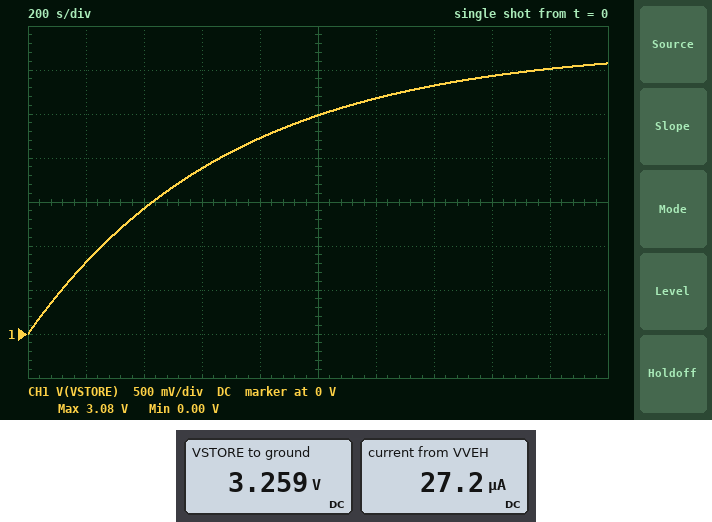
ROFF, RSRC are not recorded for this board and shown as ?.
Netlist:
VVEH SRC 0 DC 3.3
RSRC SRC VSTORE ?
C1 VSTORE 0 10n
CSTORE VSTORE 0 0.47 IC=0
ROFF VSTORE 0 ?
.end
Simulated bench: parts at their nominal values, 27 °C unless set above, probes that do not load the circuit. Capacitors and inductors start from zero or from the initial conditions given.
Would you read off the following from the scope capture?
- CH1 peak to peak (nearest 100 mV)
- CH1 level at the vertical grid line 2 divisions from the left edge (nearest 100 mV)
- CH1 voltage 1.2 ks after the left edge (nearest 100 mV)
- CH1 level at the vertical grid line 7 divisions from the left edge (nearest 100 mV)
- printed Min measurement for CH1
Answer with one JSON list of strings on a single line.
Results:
["3.1 V", "1.4 V", "2.7 V", "2.8 V", "0.00 V"]
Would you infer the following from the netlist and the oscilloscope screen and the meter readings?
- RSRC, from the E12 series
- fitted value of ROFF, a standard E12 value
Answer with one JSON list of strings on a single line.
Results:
["1.5 kΩ", "120 kΩ"]
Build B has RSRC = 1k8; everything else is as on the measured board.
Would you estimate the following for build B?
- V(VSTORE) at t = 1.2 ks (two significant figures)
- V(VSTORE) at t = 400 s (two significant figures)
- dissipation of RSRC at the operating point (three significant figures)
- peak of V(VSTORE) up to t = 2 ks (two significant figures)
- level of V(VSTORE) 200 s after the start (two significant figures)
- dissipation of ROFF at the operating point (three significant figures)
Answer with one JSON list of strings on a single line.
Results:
["2.5 V", "1.2 V", "1.32 µW", "3.0 V", "690 mV", "88.1 µW"]
